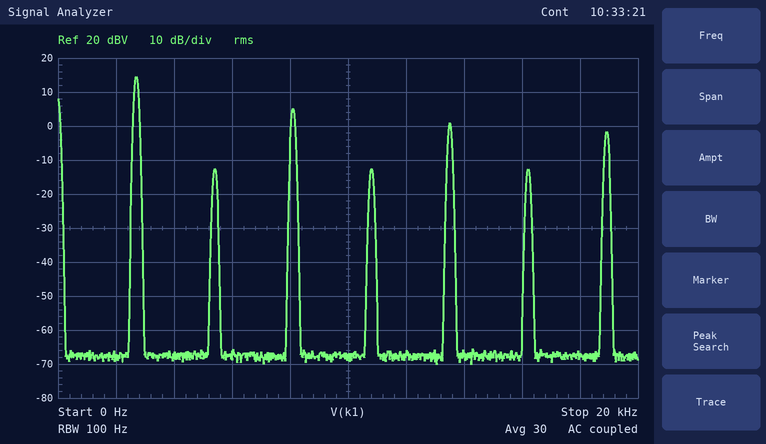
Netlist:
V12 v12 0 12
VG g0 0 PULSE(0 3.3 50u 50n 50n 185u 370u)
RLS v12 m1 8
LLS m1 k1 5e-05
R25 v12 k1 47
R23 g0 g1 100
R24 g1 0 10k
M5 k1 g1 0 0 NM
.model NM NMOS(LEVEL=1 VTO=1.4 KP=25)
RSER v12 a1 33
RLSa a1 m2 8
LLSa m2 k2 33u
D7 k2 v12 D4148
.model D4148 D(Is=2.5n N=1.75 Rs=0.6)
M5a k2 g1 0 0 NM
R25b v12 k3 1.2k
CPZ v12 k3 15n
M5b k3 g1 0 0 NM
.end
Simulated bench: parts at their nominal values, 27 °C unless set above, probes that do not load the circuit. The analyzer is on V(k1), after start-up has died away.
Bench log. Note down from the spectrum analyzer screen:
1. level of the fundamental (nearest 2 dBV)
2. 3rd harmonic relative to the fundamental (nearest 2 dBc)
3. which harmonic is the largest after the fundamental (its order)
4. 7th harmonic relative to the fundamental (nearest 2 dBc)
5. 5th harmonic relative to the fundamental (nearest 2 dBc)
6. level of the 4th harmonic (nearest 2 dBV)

14 dBV
-10 dBc
3
-16 dBc
-14 dBc
-12 dBV
